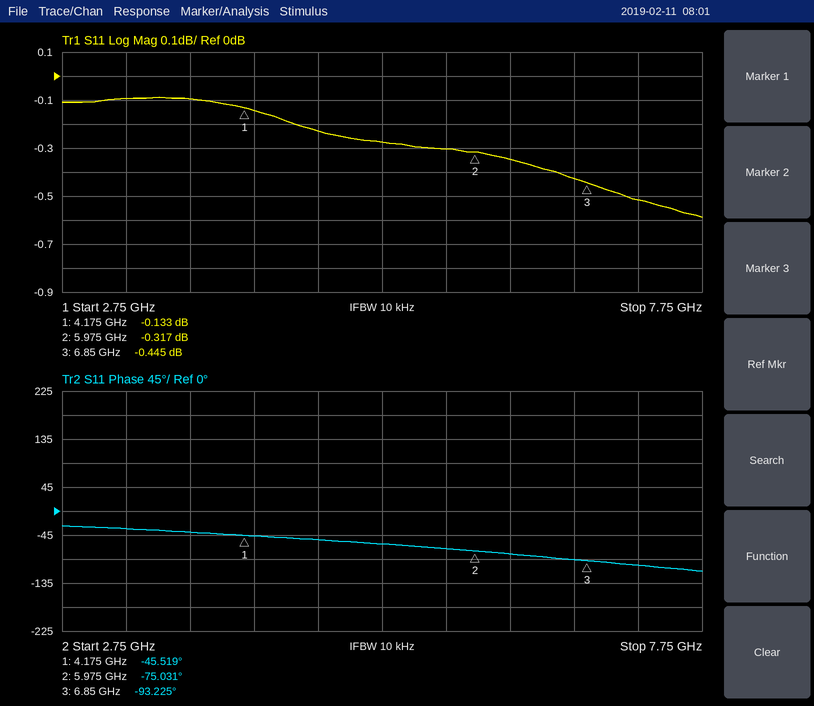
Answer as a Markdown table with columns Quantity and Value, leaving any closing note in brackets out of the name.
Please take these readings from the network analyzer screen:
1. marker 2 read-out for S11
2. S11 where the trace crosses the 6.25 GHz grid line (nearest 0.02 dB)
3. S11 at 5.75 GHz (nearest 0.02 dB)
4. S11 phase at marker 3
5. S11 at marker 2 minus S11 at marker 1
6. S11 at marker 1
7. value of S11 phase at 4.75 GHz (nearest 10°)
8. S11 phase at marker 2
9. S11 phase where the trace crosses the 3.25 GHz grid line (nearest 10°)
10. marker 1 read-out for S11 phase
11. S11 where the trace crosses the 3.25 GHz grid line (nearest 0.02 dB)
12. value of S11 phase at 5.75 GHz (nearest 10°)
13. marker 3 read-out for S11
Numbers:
| Quantity | Value |
|---|---|
| marker 2 read-out for S11 | -0.317 dB |
| S11 where the trace crosses the 6.25 GHz grid line | -0.34 dB |
| S11 at 5.75 GHz | -0.30 dB |
| S11 phase at marker 3 | -93.225° |
| S11 at marker 2 minus S11 at marker 1 | -0.184 dB |
| S11 at marker 1 | -0.133 dB |
| value of S11 phase at 4.75 GHz | -50° |
| S11 phase at marker 2 | -75.031° |
| S11 phase where the trace crosses the 3.25 GHz grid line | -30° |
| marker 1 read-out for S11 phase | -45.519° |
| S11 where the trace crosses the 3.25 GHz grid line | -0.10 dB |
| value of S11 phase at 5.75 GHz | -70° |
| marker 3 read-out for S11 | -0.445 dB |
